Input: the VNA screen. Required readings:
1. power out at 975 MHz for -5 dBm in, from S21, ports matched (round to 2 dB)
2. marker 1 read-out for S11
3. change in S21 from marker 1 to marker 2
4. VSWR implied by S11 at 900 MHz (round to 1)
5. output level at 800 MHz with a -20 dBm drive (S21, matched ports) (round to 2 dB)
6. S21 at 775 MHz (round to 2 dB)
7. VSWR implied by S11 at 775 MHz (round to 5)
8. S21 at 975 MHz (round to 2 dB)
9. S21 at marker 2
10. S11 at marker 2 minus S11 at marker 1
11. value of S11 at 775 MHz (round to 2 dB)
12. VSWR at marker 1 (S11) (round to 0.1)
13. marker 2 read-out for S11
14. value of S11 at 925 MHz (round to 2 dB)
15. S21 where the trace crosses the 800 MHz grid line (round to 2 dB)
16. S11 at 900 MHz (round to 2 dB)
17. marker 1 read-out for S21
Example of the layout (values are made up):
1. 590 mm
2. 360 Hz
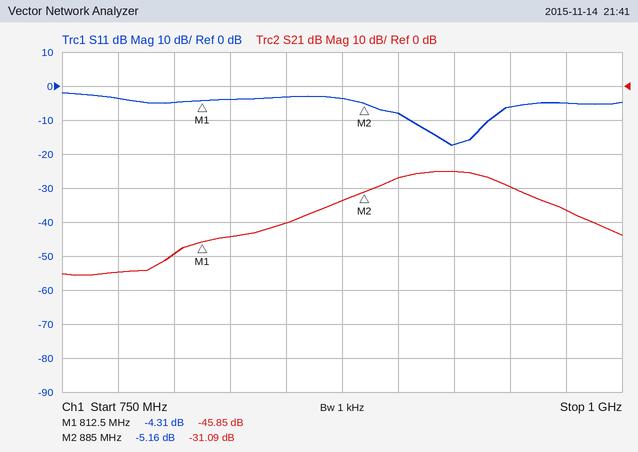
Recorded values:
1. -42 dBm
2. -4.31 dB
3. 14.76 dB
4. 2
5. -70 dBm
6. -54 dB
7. 5
8. -36 dB
9. -31.09 dB
10. -0.85 dB
11. -4 dB
12. 4.1
13. -5.16 dB
14. -18 dB
15. -50 dB
16. -8 dB
17. -45.85 dB
